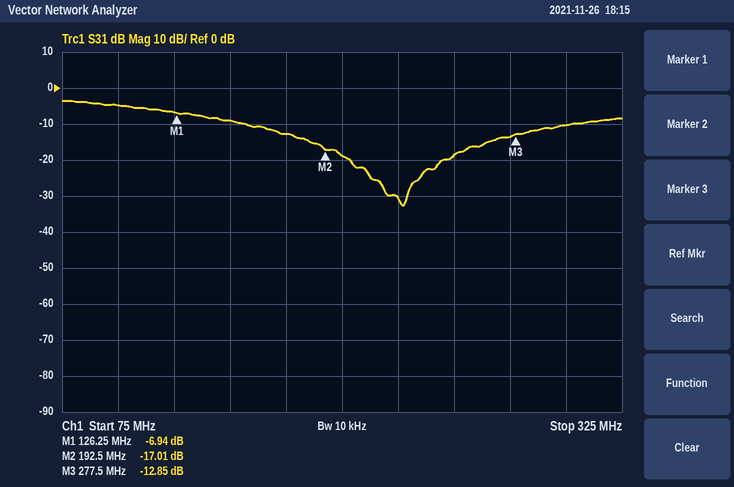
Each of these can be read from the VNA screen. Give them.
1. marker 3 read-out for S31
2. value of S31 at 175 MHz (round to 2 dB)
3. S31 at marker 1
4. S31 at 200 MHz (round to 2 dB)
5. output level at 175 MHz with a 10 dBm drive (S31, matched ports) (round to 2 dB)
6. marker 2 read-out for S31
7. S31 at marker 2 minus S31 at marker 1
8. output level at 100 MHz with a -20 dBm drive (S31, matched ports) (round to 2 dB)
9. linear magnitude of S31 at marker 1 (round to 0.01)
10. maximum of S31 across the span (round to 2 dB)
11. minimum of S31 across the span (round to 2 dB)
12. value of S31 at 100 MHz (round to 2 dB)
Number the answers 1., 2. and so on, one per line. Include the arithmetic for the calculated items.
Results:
1. -12.85 dB
2. -12 dB
3. -6.94 dB
4. -18 dB
5. 10 dBm + (-12 dB) = -2 dBm
6. -17.01 dB
7. -17.01 − (-6.94) = -10.07 dB
8. -20 dBm + (-4 dB) = -24 dBm
9. 10^(-6.94/20) ≈ 0.45
10. -4 dB
11. -32 dB
12. -4 dB
